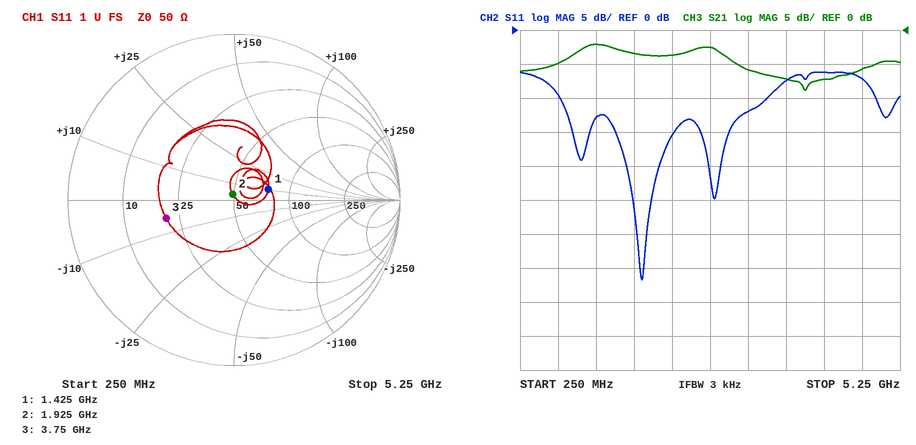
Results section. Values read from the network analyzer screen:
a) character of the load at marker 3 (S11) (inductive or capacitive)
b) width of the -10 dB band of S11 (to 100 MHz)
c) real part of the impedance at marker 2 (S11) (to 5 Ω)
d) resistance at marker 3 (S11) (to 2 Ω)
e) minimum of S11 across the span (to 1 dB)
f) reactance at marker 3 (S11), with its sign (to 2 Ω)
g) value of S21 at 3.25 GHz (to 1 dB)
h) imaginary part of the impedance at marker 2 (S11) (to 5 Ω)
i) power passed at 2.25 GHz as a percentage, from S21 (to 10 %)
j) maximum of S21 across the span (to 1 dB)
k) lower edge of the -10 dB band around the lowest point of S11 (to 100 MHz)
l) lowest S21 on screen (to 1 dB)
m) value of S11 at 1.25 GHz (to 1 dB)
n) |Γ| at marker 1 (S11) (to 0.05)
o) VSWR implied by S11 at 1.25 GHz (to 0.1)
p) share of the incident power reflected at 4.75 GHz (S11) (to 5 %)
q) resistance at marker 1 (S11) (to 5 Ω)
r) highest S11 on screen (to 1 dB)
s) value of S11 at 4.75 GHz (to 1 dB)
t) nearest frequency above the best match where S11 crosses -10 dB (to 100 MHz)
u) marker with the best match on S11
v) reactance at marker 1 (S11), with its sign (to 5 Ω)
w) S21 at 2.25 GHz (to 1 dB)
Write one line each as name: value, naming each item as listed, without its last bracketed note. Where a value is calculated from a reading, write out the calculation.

character of the load at marker 3 (S11): capacitive
width of the -10 dB band of S11: 3.5 GHz − 800 MHz = 2.7 GHz
real part of the impedance at marker 2 (S11): 50 Ω
resistance at marker 3 (S11): 20 Ω
minimum of S11 across the span: -37 dB
reactance at marker 3 (S11), with its sign: -6 Ω
value of S21 at 3.25 GHz: -6 dB
imaginary part of the impedance at marker 2 (S11): +5 Ω
power passed at 2.25 GHz as a percentage, from S21: 10^(-4/10) ≈ 40 %
maximum of S21 across the span: -2 dB
lower edge of the -10 dB band around the lowest point of S11: 800 MHz
lowest S21 on screen: -9 dB
value of S11 at 1.25 GHz: -13 dB
|Γ| at marker 1 (S11): 0.20
VSWR implied by S11 at 1.25 GHz: |Γ| = 10^(-13/20) = 0.2239; VSWR = (1 + 0.2239)/(1 − 0.2239) ≈ 1.6
share of the incident power reflected at 4.75 GHz (S11): 10^(-7/10) ≈ 20 %
resistance at marker 1 (S11): 75 Ω
highest S11 on screen: -6 dB
value of S11 at 4.75 GHz: -7 dB
nearest frequency above the best match where S11 crosses -10 dB: 3.5 GHz
marker with the best match on S11: marker 2
reactance at marker 1 (S11), with its sign: +10 Ω
S21 at 2.25 GHz: -4 dB
